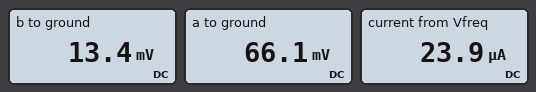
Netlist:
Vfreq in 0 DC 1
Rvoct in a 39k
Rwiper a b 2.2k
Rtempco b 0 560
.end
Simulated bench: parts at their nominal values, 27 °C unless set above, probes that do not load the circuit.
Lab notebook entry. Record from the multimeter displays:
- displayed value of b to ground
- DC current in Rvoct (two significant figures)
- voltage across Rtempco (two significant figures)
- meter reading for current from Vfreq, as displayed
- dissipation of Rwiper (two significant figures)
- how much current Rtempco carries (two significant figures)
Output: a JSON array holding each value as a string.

["13.4 mV", "24 µA", "13 mV", "23.9 µA", "1.3 µW", "24 µA"]
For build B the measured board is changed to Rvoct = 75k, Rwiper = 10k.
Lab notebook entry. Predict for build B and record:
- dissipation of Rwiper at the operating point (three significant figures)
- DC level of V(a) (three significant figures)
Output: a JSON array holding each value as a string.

["1.37 µW", "123 mV"]
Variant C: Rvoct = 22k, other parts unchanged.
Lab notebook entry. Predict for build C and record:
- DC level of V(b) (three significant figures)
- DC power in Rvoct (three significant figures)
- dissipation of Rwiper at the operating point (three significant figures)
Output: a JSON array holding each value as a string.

["22.6 mV", "35.9 µW", "3.59 µW"]
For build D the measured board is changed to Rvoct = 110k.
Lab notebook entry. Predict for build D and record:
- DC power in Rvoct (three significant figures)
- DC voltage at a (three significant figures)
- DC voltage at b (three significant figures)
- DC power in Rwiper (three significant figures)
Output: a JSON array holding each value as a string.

["8.65 µW", "24.5 mV", "4.97 mV", "173 nW"]
